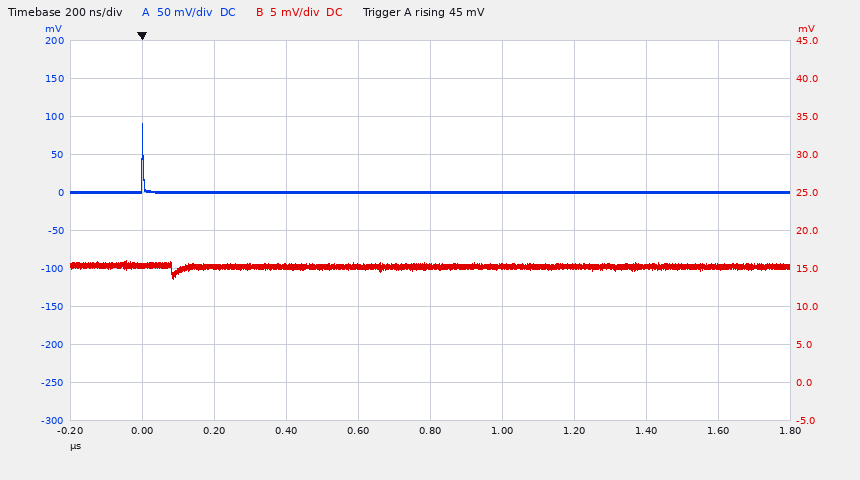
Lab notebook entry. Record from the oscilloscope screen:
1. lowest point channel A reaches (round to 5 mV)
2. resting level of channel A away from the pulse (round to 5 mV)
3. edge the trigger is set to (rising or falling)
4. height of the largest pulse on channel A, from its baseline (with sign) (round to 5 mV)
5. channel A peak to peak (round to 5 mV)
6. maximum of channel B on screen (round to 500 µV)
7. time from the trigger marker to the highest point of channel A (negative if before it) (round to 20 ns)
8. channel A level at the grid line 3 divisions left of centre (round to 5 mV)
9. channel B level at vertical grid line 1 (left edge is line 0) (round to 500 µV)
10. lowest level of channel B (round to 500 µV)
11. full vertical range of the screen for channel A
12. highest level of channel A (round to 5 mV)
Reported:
0 mV
0 mV
rising
+90 mV
90 mV
16.0 mV
0 ns
0 mV
15.5 mV
13.5 mV
500 mV
90 mV
